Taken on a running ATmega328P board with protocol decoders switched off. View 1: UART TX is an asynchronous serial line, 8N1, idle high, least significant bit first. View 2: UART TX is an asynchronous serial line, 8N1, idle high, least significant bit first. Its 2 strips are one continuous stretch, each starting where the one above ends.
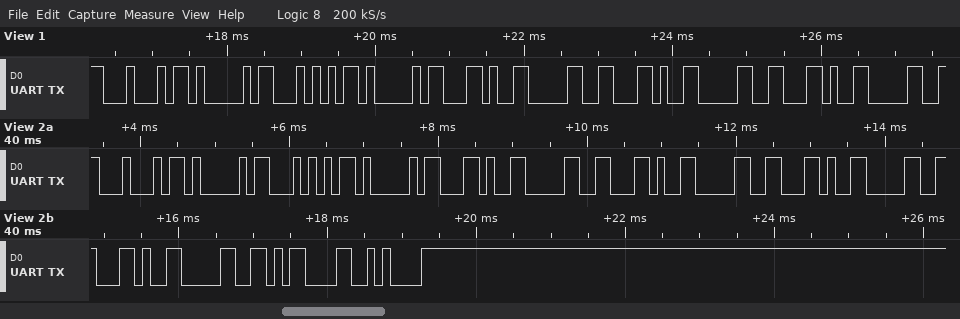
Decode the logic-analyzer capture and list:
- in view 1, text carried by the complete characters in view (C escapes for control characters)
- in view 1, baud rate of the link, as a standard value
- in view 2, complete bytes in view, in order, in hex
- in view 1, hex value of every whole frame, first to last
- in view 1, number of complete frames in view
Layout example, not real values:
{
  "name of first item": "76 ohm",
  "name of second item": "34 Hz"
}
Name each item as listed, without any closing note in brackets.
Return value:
{
  "in view 1, text carried by the complete characters in view": "\"DATA,0,0,0\"",
  "in view 1, baud rate of the link, as a standard value": "9600 baud",
  "in view 2, complete bytes in view, in order, in hex": "44 41 54 41 2C 30 2C 30 2C 30 2C 30 0D 0A",
  "in view 1, hex value of every whole frame, first to last": "44 41 54 41 2C 30 2C 30 2C 30",
  "in view 1, number of complete frames in view": "10"
}
